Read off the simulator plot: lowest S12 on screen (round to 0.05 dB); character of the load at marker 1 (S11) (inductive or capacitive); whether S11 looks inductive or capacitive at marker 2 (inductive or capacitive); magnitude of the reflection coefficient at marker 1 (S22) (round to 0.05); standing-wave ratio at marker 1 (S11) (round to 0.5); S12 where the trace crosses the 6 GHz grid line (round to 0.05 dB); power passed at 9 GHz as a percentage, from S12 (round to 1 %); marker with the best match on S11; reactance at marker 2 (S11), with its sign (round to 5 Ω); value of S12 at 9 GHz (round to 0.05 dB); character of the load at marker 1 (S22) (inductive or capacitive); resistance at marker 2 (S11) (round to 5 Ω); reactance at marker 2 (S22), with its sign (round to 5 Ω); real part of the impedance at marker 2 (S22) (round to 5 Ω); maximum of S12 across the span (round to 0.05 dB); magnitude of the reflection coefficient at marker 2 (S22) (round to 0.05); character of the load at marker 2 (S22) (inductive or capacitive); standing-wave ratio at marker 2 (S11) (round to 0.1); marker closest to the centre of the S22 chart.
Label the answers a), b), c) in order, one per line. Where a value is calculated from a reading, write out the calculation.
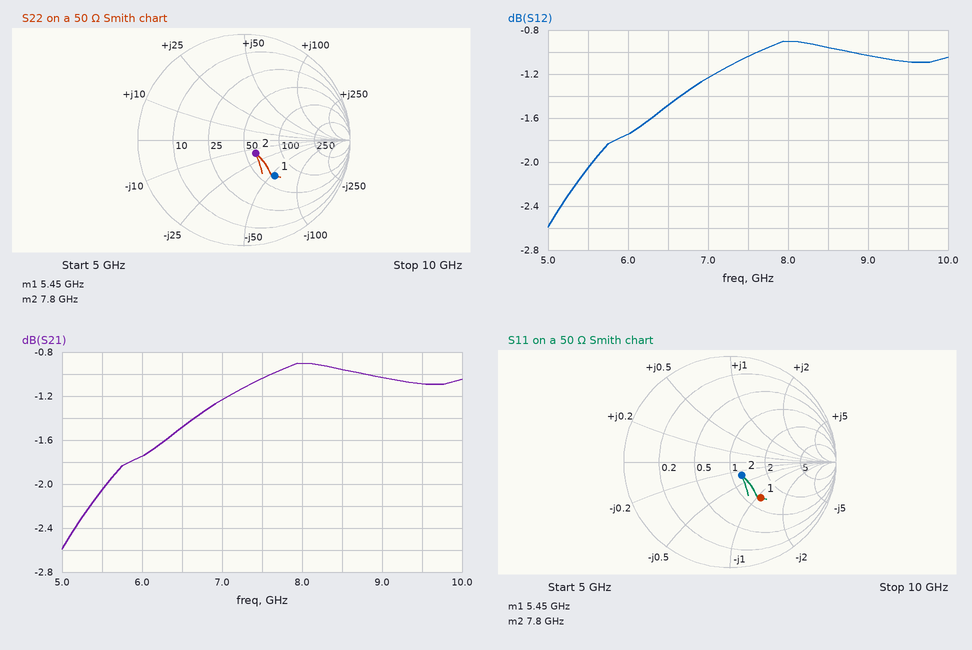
a) -2.60 dB
b) capacitive
c) capacitive
d) 0.45
e) 2.5
f) -1.75 dB
g) 10^(-1.05/10) ≈ 79 %
h) marker 2
i) -15 Ω
j) -1.05 dB
k) capacitive
l) 60 Ω
m) -15 Ω
n) 60 Ω
o) -0.90 dB
p) 0.15
q) capacitive
r) 1.4
s) marker 2
